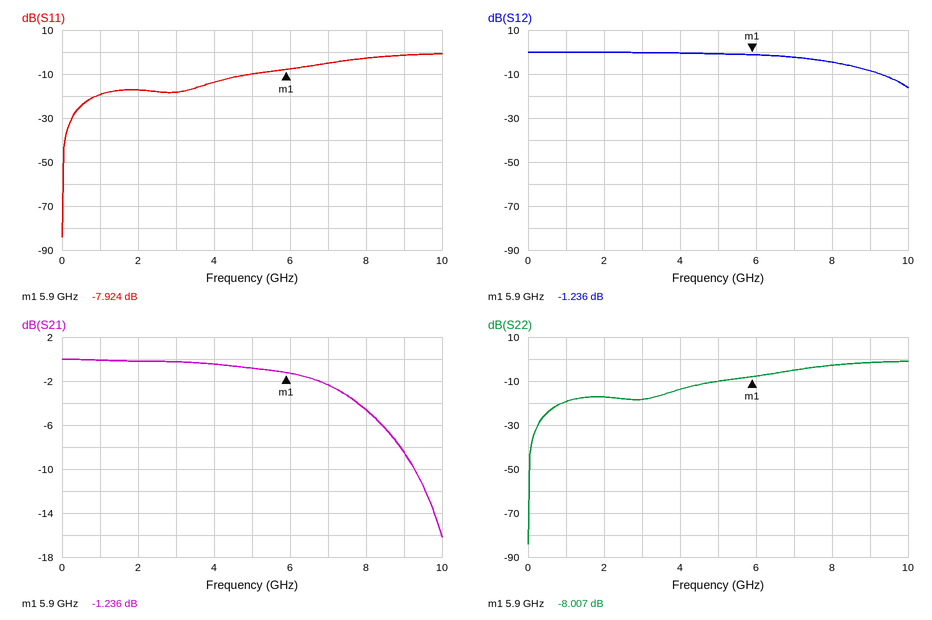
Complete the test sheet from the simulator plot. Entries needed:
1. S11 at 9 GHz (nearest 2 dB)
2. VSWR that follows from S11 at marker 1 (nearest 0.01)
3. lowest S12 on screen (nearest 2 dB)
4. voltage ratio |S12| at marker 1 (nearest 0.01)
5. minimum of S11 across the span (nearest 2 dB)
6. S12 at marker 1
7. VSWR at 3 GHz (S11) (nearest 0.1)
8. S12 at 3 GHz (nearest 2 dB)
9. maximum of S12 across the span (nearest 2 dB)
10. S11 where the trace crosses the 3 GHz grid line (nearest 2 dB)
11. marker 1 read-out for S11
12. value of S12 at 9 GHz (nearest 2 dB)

-2 dB
2.34
-16 dB
0.87
-84 dB
-1.236 dB
1.3
0 dB
0 dB
-18 dB
-7.924 dB
-8 dB
